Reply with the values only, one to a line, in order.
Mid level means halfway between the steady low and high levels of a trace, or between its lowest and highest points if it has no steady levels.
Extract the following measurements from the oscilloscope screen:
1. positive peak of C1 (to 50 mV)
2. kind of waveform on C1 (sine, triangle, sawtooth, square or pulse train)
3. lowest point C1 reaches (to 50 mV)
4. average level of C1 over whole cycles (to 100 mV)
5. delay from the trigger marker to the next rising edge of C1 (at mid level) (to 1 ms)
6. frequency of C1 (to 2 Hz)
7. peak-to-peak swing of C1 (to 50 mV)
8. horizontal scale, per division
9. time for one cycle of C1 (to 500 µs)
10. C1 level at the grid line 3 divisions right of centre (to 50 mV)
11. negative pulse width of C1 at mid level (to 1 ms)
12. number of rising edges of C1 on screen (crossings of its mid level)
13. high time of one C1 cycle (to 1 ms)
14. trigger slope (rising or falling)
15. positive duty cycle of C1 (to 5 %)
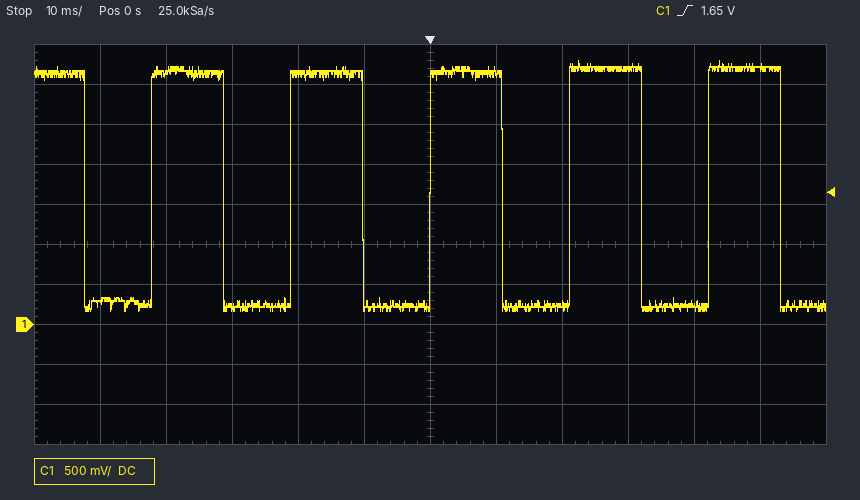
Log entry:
3.30 V
square
200 mV
1.8 V
21 ms
48 Hz
3.10 V
10 ms
21.0 ms
3.20 V
10 ms
5
11 ms
rising
50 %
